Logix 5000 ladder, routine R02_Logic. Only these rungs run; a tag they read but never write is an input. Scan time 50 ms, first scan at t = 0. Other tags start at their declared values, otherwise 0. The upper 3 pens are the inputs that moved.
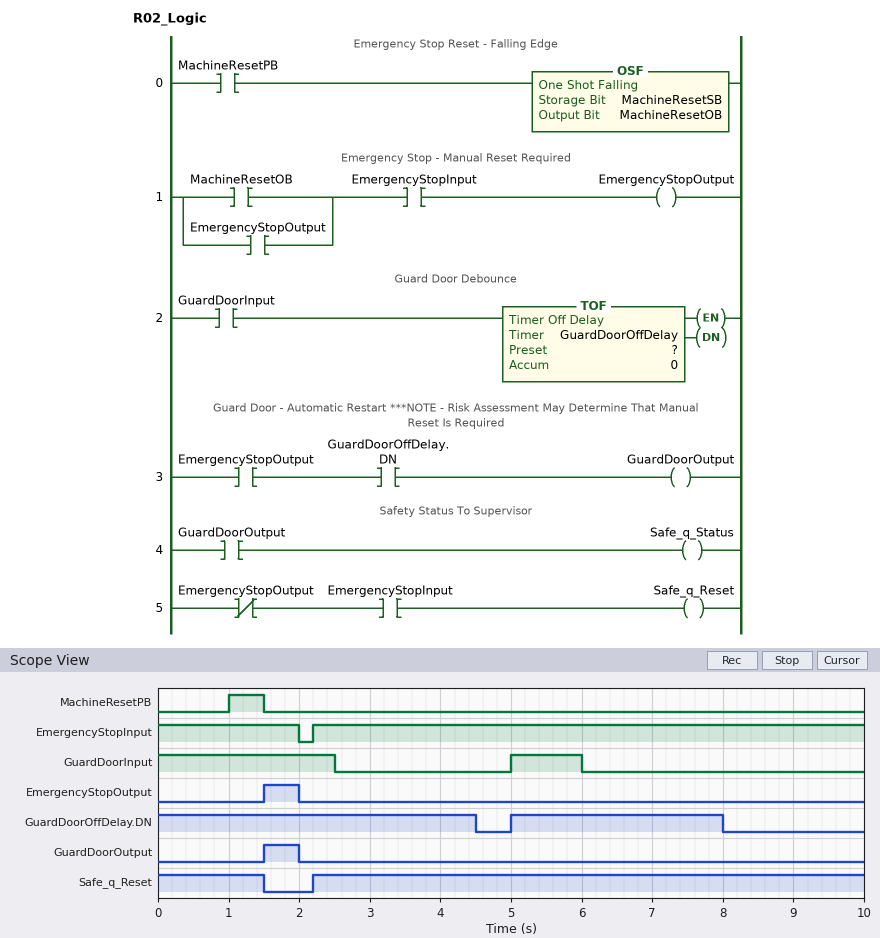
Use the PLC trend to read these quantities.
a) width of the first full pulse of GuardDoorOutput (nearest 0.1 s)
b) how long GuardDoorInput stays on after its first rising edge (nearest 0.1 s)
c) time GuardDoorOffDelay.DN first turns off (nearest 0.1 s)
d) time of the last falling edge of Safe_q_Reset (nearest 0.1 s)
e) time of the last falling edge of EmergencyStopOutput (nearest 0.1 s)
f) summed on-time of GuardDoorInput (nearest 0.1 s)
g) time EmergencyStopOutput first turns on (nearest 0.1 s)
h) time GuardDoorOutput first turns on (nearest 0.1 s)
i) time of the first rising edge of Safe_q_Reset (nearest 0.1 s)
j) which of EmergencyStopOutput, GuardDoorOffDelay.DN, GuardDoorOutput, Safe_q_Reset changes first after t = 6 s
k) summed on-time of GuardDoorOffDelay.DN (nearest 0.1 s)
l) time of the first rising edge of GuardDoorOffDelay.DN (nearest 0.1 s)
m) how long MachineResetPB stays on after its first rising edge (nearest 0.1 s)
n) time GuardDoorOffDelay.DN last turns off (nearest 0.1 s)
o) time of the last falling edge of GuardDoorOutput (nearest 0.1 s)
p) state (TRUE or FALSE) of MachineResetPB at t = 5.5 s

0.5 s
1.0 s
4.5 s
1.5 s
2.0 s
3.5 s
1.5 s
1.5 s
2.2 s
GuardDoorOffDelay.DN
7.5 s
5.0 s
0.5 s
8.0 s
2.0 s
FALSE
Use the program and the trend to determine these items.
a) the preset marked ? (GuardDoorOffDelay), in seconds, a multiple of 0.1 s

2.0 s
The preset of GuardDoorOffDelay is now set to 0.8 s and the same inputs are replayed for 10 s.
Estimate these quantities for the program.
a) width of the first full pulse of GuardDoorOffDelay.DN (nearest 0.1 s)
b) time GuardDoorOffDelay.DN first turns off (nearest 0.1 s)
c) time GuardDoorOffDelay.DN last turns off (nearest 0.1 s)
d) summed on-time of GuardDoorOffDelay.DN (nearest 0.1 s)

1.8 s
3.3 s
6.8 s
5.1 s
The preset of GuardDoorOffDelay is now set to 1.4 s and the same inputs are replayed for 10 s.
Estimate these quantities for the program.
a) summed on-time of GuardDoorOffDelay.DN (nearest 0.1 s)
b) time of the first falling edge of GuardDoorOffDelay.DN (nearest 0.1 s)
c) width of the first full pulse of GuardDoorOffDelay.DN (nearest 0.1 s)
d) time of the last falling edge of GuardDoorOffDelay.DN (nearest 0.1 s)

6.3 s
3.9 s
2.4 s
7.4 s
